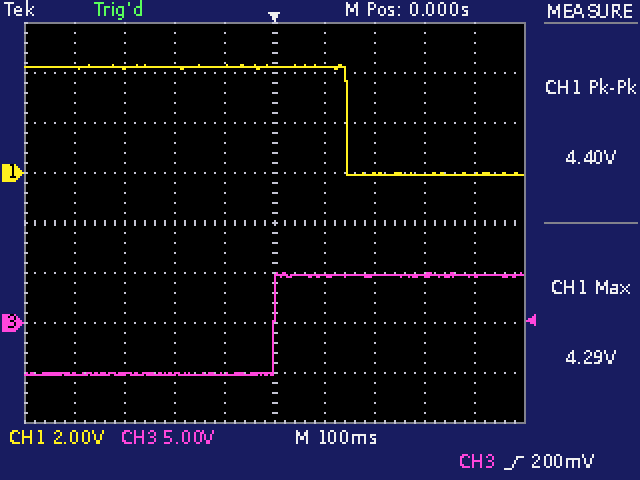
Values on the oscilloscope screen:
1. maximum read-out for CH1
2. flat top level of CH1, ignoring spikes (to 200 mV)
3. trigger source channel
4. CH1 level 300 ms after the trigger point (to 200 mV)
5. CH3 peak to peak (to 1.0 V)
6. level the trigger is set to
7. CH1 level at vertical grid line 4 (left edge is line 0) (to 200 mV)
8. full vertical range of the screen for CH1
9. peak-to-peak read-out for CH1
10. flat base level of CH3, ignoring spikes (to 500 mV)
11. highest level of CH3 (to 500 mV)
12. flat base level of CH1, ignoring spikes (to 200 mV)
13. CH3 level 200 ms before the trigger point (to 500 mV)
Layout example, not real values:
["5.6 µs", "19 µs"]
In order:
["4.29 V", "4.2 V", "CH3", "0.0 V", "10.0 V", "200 mV", "4.2 V", "16 V", "4.40 V", "-5.0 V", "5.0 V", "0.0 V", "-5.0 V"]
